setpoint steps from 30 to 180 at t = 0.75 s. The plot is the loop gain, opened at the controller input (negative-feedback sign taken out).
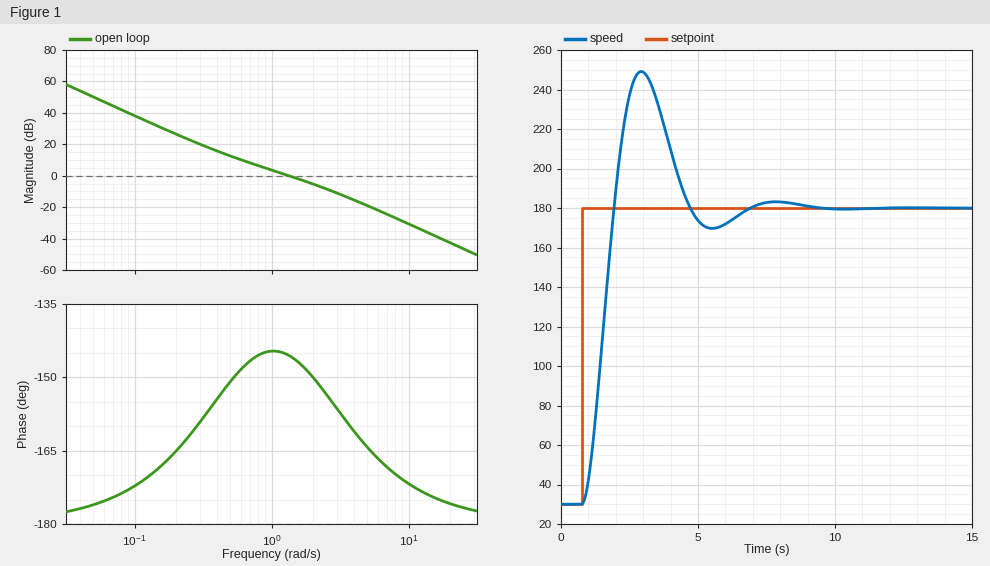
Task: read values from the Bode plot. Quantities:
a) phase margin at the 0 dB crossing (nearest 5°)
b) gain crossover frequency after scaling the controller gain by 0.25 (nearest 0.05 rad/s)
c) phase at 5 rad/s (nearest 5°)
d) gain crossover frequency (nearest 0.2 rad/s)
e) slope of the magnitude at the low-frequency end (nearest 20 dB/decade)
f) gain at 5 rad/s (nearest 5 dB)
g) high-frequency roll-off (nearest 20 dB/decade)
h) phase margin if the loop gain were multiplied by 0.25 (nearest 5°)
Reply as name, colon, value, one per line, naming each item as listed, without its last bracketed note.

phase margin at the 0 dB crossing: 35°
gain crossover frequency after scaling the controller gain by 0.25: 0.50 rad/s
phase at 5 rad/s: -165°
gain crossover frequency: 1.4 rad/s
slope of the magnitude at the low-frequency end: -40 dB/decade
gain at 5 rad/s: -20 dB
high-frequency roll-off: -40 dB/decade
phase margin if the loop gain were multiplied by 0.25: 30°
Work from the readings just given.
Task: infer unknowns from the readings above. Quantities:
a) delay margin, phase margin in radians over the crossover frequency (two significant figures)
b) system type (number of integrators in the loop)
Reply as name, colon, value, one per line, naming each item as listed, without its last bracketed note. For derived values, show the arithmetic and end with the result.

delay margin, phase margin in radians over the crossover frequency: 35 × π / 180 / 1.4 = 0.44 s
system type: 2
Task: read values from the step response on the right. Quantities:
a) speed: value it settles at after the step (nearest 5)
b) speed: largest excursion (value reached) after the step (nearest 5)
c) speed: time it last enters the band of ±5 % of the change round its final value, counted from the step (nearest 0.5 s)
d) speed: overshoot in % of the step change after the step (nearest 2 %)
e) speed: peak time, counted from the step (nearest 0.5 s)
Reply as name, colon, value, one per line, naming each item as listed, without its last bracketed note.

speed: value it settles at after the step: 180
speed: largest excursion (value reached) after the step: 250
speed: time it last enters the band of ±5 % of the change round its final value, counted from the step: 5.5 s
speed: overshoot in % of the step change after the step: 46 %
speed: peak time, counted from the step: 2.0 s
